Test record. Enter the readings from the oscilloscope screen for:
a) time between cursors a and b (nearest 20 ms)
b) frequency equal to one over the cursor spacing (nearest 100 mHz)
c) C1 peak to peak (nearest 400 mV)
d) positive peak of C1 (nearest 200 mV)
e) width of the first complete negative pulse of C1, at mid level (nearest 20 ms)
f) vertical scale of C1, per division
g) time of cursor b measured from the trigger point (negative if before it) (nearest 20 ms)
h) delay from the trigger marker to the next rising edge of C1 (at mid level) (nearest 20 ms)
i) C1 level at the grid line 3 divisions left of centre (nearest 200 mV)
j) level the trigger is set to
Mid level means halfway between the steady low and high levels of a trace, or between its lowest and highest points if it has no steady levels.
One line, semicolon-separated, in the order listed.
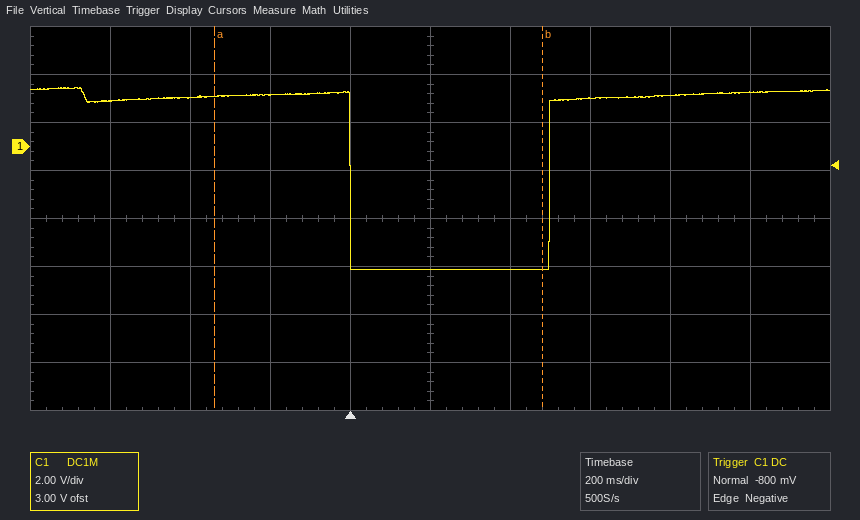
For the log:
820 ms; 1.2 Hz; 7.6 V; 2.4 V; 500 ms; 2 V; +480 ms; 500 ms; 2.0 V; -800 mV
